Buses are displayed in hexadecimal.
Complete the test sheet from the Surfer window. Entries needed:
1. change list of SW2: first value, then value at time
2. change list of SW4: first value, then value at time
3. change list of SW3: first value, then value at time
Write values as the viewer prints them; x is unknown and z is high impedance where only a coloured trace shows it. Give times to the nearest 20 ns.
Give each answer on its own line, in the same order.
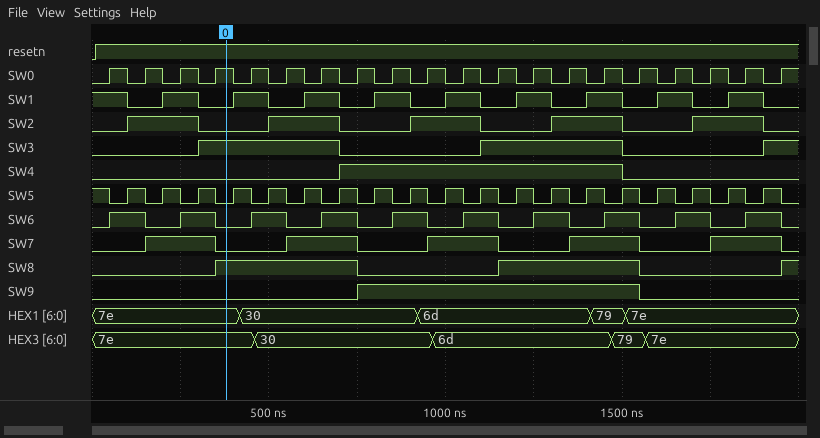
0, 1 at 100 ns, 0 at 300 ns, 1 at 500 ns, 0 at 700 ns, 1 at 900 ns, 0 at 1100 ns, 1 at 1300 ns, 0 at 1500 ns, 1 at 1700 ns, 0 at 1900 ns
0, 1 at 700 ns, 0 at 1500 ns
0, 1 at 300 ns, 0 at 700 ns, 1 at 1100 ns, 0 at 1500 ns, 1 at 1900 ns
